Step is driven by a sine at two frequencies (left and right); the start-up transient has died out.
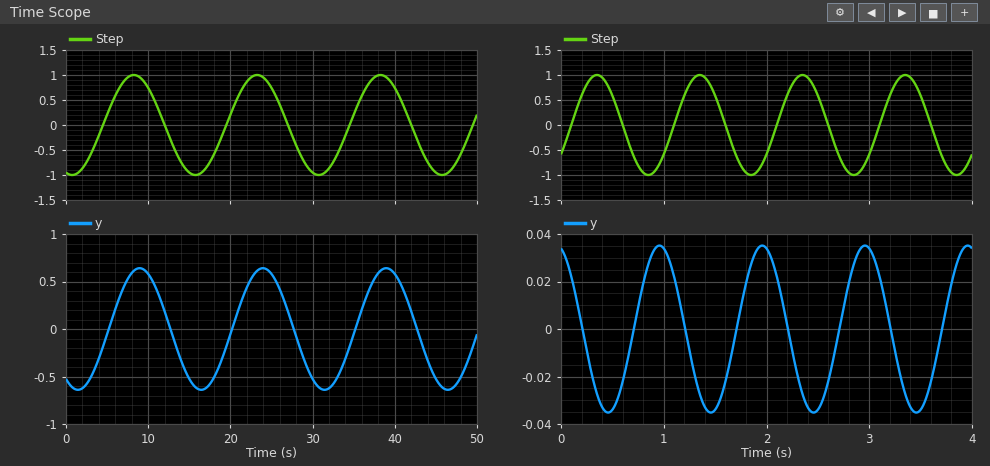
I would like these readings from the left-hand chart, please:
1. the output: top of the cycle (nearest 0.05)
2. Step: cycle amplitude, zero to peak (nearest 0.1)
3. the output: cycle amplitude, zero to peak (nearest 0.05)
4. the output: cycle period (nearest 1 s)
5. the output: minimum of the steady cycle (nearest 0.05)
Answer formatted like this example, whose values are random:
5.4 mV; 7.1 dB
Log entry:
0.65; 1.0; 0.65; 15 s; -0.65
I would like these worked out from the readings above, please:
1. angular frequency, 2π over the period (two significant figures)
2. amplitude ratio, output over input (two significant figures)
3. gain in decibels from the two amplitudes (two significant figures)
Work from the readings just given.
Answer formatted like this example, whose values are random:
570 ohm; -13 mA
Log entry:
0.42 rad/s; 0.65; -3.7 dB
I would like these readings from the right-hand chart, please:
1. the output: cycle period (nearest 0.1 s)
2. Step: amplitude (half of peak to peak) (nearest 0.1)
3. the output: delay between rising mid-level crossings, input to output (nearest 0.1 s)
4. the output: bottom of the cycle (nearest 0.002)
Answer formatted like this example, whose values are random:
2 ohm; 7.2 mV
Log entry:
1.0 s; 1.0; 0.6 s; -0.036
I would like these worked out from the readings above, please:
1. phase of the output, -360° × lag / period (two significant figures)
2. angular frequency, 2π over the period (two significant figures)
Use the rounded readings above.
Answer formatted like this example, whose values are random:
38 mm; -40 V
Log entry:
-220°; 6.3 rad/s
